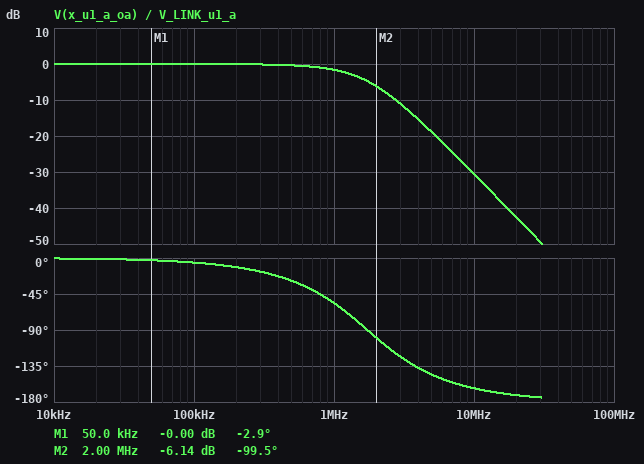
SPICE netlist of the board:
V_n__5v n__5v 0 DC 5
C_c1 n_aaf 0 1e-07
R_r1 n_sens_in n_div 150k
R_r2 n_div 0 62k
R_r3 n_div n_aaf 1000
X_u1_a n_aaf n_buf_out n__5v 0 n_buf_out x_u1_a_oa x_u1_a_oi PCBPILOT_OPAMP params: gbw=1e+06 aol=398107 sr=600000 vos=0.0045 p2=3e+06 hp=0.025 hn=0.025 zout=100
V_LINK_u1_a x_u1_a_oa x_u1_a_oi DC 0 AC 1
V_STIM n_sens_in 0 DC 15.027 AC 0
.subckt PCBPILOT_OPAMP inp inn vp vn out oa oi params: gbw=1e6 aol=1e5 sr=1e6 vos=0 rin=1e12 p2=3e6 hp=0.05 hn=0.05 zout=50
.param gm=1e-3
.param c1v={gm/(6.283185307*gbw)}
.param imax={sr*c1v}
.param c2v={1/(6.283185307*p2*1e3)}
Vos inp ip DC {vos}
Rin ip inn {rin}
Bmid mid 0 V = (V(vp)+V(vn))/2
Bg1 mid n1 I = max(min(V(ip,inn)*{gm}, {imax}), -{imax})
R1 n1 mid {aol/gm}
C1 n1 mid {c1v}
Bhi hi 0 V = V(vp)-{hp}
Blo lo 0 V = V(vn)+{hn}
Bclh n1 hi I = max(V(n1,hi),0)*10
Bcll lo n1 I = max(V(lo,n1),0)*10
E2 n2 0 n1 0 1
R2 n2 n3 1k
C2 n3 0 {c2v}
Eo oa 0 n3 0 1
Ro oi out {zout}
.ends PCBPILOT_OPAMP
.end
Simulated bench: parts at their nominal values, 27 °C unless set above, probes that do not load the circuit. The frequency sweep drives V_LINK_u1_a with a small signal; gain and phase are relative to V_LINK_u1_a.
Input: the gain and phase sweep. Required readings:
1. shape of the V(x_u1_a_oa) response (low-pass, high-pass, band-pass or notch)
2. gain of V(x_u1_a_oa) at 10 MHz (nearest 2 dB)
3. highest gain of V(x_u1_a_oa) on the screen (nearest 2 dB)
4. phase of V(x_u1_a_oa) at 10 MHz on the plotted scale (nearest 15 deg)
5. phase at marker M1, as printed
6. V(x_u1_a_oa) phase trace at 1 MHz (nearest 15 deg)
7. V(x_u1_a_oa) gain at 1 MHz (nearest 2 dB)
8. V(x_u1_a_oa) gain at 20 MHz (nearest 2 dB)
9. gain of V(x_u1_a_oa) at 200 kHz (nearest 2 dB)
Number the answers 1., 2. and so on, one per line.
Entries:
1. low-pass
2. -30 dB
3. 0 dB
4. -165 deg
5. -2.9 deg
6. -60 deg
7. -2 dB
8. -42 dB
9. 0 dB
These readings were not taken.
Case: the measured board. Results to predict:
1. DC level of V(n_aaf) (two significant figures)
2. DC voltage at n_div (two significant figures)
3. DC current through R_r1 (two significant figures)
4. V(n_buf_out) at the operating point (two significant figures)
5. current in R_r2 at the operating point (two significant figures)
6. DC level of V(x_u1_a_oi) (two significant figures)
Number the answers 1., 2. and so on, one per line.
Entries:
1. 4.4 V
2. 4.4 V
3. 71 µA
4. 4.4 V
5. 71 µA
6. 4.4 V
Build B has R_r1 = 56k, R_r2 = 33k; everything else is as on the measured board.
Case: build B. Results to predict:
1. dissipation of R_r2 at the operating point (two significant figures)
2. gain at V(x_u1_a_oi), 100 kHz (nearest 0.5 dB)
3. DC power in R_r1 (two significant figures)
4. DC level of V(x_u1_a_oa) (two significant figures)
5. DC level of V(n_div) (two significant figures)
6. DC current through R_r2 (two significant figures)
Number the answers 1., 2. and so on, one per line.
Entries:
1. 940 µW
2. 0 dB
3. 1.6 mW
4. 5.0 V
5. 5.6 V
6. 170 µA
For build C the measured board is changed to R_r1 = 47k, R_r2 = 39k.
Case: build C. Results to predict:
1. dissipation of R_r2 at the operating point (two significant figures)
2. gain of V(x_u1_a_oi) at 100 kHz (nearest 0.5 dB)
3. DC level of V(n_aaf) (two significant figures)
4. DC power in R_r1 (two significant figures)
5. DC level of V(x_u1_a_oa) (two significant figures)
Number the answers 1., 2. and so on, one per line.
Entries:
1. 1.2 mW
2. 0 dB
3. 6.8 V
4. 1.4 mW
5. 5.0 V
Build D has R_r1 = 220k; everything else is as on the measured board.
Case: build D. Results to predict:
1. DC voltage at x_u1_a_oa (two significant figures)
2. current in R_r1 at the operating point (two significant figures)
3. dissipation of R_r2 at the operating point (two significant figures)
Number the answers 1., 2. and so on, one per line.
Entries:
1. 3.3 V
2. 53 µA
3. 180 µW
